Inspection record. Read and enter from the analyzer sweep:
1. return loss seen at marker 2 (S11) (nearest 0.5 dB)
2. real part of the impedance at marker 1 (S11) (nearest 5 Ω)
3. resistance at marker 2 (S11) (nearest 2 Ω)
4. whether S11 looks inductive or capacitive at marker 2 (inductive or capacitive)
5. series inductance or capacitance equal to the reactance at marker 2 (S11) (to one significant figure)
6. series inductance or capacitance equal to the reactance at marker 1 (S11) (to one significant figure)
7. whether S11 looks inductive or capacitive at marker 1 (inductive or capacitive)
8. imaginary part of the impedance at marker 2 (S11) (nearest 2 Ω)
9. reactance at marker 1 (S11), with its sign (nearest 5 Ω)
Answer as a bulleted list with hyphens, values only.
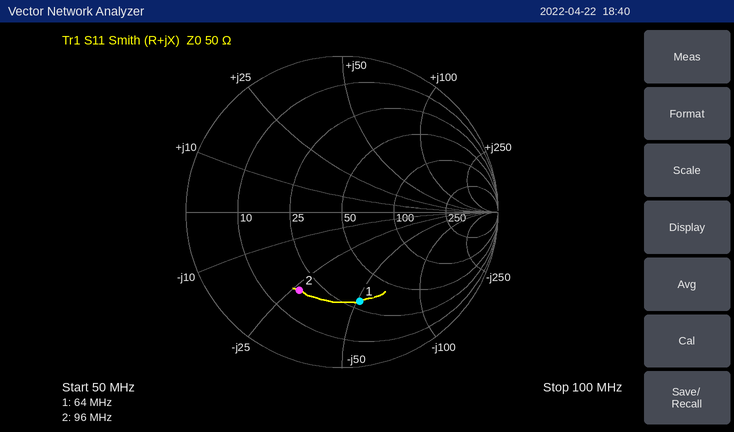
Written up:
- 5.0 dB
- 30 Ω
- 18 Ω
- capacitive
- 60 pF
- 50 pF
- capacitive
- -26 Ω
- -50 Ω
